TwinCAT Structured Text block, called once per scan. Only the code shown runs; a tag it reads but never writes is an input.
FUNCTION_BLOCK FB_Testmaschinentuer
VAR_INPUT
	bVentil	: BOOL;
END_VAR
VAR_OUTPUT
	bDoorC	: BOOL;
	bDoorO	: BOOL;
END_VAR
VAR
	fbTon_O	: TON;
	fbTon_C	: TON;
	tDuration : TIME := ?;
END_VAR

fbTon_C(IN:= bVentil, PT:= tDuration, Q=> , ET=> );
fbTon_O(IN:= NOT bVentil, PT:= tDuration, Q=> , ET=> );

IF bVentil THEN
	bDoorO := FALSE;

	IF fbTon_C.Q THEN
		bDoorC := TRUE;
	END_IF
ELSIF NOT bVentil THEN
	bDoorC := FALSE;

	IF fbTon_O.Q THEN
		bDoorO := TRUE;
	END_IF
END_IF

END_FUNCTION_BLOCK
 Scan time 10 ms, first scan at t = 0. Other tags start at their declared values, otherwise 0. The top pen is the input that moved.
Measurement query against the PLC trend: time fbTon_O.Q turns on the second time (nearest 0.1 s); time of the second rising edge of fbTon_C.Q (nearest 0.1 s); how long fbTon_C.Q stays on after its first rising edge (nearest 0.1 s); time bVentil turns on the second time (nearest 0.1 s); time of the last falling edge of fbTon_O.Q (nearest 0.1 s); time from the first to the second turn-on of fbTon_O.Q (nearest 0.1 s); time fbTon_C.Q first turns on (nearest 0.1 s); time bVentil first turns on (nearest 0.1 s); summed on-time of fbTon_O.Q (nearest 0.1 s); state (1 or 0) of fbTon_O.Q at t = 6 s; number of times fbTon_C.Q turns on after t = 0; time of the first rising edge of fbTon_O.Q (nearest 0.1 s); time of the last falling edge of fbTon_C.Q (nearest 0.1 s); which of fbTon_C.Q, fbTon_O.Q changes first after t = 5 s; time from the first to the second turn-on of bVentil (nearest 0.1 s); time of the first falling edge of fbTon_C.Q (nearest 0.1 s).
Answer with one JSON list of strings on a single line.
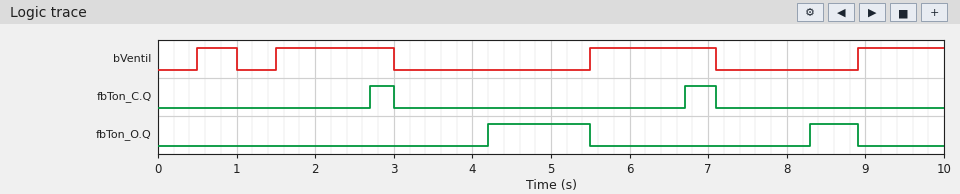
["8.3 s", "6.7 s", "0.3 s", "1.5 s", "8.9 s", "4.1 s", "2.7 s", "0.5 s", "1.9 s", "0", "2", "4.2 s", "7.1 s", "fbTon_O.Q", "1.0 s", "3.0 s"]
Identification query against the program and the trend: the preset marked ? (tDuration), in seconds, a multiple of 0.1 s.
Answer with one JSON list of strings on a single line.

["1.2 s"]
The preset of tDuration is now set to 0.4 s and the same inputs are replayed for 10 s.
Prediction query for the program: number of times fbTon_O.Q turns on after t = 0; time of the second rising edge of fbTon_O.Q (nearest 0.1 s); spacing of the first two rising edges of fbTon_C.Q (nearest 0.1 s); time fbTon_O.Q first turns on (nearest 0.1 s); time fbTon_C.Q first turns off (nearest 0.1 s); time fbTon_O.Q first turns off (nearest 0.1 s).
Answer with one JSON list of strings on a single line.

["4", "1.4 s", "1.0 s", "0.4 s", "1.0 s", "0.5 s"]
